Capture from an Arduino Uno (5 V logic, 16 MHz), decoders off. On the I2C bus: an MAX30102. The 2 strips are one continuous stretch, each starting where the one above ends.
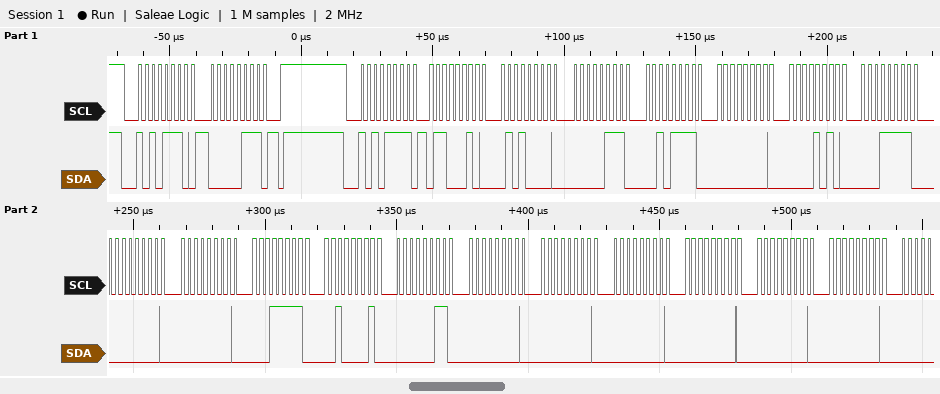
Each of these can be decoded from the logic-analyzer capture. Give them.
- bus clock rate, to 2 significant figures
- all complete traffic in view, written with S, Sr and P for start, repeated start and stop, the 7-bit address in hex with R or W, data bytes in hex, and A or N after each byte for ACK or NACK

400 kHz
S 57W A 07 A P S 57R A 62 A 50 A 07 A 2F A 00 A 0A A 1F A 00 A 00 A 1F A 21 A 03 A 00 A 00 A 00 A 00 A 00 A 00 A
